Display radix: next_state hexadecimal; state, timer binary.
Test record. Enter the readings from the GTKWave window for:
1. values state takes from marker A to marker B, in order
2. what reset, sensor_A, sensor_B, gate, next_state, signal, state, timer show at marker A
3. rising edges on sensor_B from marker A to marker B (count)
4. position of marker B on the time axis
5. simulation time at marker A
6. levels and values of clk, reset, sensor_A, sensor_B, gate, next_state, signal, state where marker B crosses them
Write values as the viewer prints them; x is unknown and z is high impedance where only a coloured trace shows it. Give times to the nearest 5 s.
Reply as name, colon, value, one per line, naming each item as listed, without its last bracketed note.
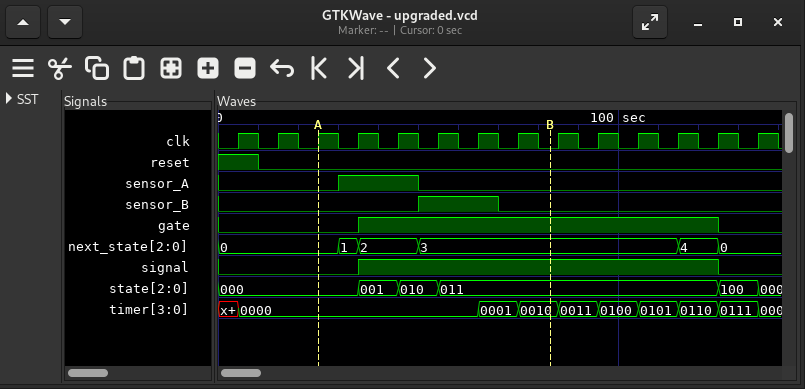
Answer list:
values state takes from marker A to marker B, in order: 000, 001, 010, 011
what reset, sensor_A, sensor_B, gate, next_state, signal, state, timer show at marker A: reset=0, sensor_A=0, sensor_B=0, gate=0, next_state=0, signal=0, state=000, timer=0000
rising edges on sensor_B from marker A to marker B: 1
position of marker B on the time axis: 85 s
simulation time at marker A: 25 s
levels and values of clk, reset, sensor_A, sensor_B, gate, next_state, signal, state where marker B crosses them: clk=0, reset=0, sensor_A=0, sensor_B=0, gate=1, next_state=3, signal=1, state=011
